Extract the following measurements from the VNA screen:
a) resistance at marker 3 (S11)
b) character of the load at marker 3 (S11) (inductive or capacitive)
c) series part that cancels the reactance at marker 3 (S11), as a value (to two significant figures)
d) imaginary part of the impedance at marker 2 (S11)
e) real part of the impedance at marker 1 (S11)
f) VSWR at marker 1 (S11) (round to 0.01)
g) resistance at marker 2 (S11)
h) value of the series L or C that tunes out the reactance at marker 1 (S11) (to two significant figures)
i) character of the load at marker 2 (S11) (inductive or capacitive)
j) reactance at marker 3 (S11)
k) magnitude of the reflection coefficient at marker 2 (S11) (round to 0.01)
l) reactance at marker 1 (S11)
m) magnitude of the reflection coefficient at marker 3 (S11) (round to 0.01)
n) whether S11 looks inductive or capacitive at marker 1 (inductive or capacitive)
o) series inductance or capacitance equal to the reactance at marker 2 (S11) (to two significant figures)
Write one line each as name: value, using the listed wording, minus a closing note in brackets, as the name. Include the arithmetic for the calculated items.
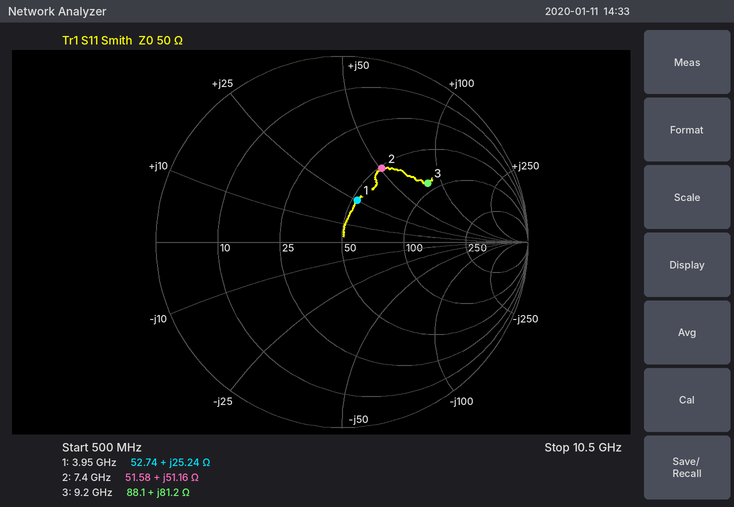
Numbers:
resistance at marker 3: 88.1 Ω
character of the load at marker 3 (S11): inductive
series part that cancels the reactance at marker 3 (S11), as a value: C = 1/(2π × 9.2 GHz × 81.2 Ω) ≈ 213 fF, so 210 fF to two significant figures
imaginary part of the impedance at marker 2: +51.16 Ω
real part of the impedance at marker 1: 52.74 Ω
VSWR at marker 1 (S11): 1.63
resistance at marker 2: 51.58 Ω
value of the series L or C that tunes out the reactance at marker 1 (S11): C = 1/(2π × 3.95 GHz × 25.24 Ω) ≈ 1.6 pF
character of the load at marker 2 (S11): inductive
reactance at marker 3: +81.2 Ω
magnitude of the reflection coefficient at marker 2 (S11): 0.45
reactance at marker 1: +25.24 Ω
magnitude of the reflection coefficient at marker 3 (S11): 0.56
whether S11 looks inductive or capacitive at marker 1: inductive
series inductance or capacitance equal to the reactance at marker 2 (S11): L = 51.16 Ω/(2π × 7.4 GHz) ≈ 1.1 nH
